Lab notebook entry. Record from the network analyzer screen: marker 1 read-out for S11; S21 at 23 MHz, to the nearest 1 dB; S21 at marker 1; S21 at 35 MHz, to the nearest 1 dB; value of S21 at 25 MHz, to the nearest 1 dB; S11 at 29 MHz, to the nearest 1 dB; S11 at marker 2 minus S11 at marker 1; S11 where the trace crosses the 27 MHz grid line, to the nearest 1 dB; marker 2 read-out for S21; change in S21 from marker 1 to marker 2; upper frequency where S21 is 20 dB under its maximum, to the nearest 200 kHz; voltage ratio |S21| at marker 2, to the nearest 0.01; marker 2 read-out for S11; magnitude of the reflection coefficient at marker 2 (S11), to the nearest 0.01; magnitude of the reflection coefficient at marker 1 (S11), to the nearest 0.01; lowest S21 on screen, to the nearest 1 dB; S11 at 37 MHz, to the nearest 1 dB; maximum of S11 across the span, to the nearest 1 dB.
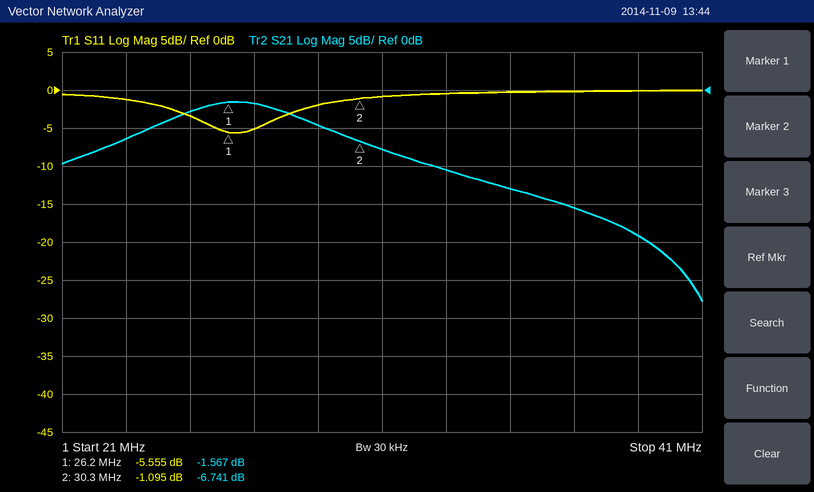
-5.555 dB
-6 dB
-1.567 dB
-13 dB
-3 dB
-2 dB
4.460 dB
-5 dB
-6.741 dB
-5.174 dB
39.8 MHz
0.46
-1.095 dB
0.88
0.53
-28 dB
0 dB
0 dB
